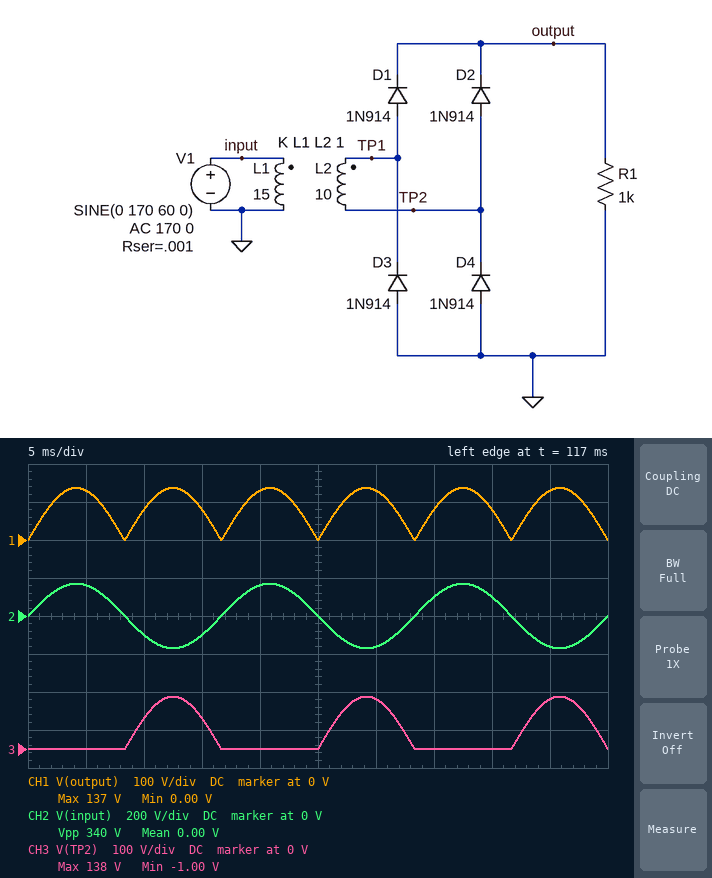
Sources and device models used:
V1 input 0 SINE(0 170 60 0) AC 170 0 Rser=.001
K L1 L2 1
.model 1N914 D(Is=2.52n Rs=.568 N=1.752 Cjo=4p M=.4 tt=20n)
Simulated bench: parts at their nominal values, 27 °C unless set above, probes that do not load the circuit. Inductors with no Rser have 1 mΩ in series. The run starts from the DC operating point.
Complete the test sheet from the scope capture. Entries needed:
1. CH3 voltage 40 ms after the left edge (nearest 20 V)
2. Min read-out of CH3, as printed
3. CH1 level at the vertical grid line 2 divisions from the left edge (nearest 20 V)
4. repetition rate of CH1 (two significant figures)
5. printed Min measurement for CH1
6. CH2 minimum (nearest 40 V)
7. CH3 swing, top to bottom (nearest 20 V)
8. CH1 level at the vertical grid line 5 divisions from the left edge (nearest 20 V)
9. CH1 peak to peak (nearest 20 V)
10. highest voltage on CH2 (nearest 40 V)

0 V
-1.00 V
80 V
120 Hz
0.00 V
-160 V
140 V
0 V
140 V
160 V
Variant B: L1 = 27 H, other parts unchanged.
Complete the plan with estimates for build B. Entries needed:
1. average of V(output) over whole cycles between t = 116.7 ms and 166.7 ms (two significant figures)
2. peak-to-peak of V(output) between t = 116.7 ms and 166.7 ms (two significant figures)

64 V
100 V
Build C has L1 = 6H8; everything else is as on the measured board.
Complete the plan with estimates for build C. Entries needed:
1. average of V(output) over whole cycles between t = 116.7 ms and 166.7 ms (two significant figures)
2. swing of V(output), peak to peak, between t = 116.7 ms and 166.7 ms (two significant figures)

130 V
200 V
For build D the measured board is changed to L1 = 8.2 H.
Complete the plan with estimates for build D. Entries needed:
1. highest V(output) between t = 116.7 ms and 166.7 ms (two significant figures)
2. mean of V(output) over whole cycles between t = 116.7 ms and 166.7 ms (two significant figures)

190 V
120 V
